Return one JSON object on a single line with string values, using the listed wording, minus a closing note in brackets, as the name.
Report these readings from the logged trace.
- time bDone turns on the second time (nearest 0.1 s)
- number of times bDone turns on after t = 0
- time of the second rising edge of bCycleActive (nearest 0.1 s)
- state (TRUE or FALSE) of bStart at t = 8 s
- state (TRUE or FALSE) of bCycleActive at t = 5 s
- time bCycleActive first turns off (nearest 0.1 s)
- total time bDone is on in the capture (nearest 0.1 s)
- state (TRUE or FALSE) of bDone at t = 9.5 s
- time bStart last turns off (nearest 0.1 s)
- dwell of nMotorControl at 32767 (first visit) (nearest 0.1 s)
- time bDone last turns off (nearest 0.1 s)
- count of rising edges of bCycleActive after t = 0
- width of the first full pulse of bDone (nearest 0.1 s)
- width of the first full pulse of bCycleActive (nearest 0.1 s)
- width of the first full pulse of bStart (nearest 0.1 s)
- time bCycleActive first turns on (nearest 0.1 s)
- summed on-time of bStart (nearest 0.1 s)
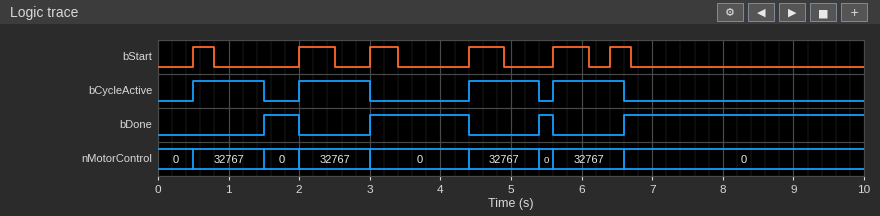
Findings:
{"time bDone turns on the second time": "3.0 s", "number of times bDone turns on after t = 0": "4", "time of the second rising edge of bCycleActive": "2.0 s", "state (TRUE or FALSE) of bStart at t = 8 s": "FALSE", "state (TRUE or FALSE) of bCycleActive at t = 5 s": "TRUE", "time bCycleActive first turns off": "1.5 s", "total time bDone is on in the capture": "5.5 s", "state (TRUE or FALSE) of bDone at t = 9.5 s": "TRUE", "time bStart last turns off": "6.7 s", "dwell of nMotorControl at 32767 (first visit)": "1.0 s", "time bDone last turns off": "5.6 s", "count of rising edges of bCycleActive after t = 0": "4", "width of the first full pulse of bDone": "0.5 s", "width of the first full pulse of bCycleActive": "1.0 s", "width of the first full pulse of bStart": "0.3 s", "time bCycleActive first turns on": "0.5 s", "summed on-time of bStart": "2.5 s"}
